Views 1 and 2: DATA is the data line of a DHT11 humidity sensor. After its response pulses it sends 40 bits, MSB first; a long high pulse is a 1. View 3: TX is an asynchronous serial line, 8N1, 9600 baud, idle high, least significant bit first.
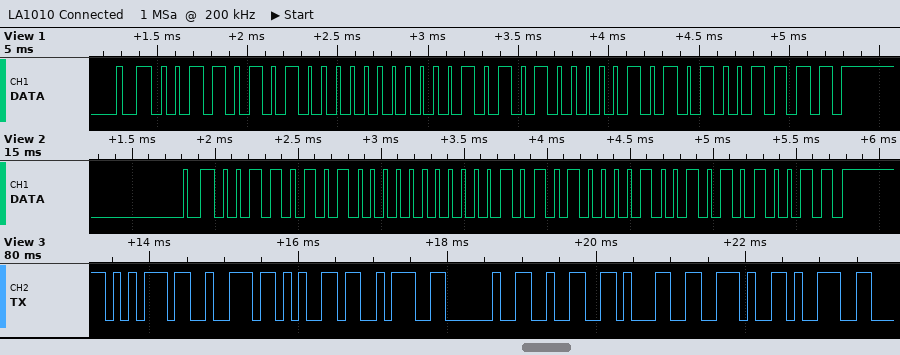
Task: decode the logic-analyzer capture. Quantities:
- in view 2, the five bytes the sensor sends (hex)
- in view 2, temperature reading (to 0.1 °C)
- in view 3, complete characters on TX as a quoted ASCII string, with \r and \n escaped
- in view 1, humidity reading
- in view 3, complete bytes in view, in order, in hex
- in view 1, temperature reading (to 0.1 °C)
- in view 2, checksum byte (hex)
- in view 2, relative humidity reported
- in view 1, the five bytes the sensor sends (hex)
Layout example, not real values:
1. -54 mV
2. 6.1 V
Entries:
1. 35 00 15 09 53
2. 21.9 °C
3. "ure: 21.9"
4. 53 %
5. 75 72 65 3A 20 32 31 2E 39
6. 21.5 °C
7. 0x53
8. 53 %
9. 35 00 15 05 4F
